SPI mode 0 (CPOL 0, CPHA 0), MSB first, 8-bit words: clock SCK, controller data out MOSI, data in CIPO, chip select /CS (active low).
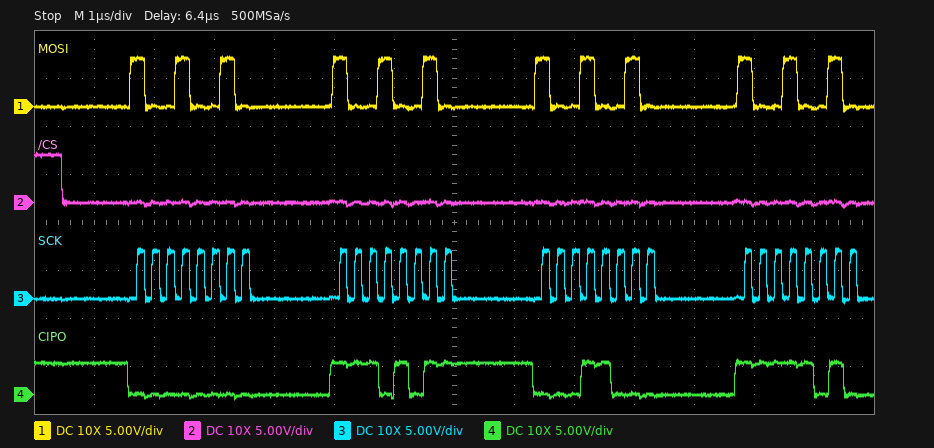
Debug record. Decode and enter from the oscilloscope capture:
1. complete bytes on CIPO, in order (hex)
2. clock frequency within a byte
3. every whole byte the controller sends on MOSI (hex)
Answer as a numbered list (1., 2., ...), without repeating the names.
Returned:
1. 00 EB 18 FA
2. 4 MHz
3. 92 92 92 92
